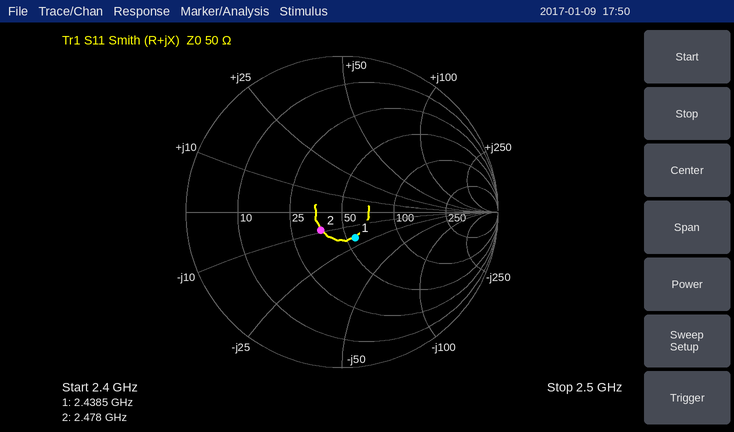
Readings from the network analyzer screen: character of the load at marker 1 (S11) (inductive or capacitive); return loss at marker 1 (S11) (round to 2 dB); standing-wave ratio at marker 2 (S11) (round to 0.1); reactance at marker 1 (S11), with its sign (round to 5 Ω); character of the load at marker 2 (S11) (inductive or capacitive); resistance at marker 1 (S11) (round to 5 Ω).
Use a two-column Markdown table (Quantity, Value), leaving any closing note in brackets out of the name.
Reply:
| Quantity | Value |
|---|---|
| character of the load at marker 1 (S11) | capacitive |
| return loss at marker 1 (S11) | 14 dB |
| standing-wave ratio at marker 2 (S11) | 1.4 |
| reactance at marker 1 (S11), with its sign | -20 Ω |
| character of the load at marker 2 (S11) | capacitive |
| resistance at marker 1 (S11) | 55 Ω |
